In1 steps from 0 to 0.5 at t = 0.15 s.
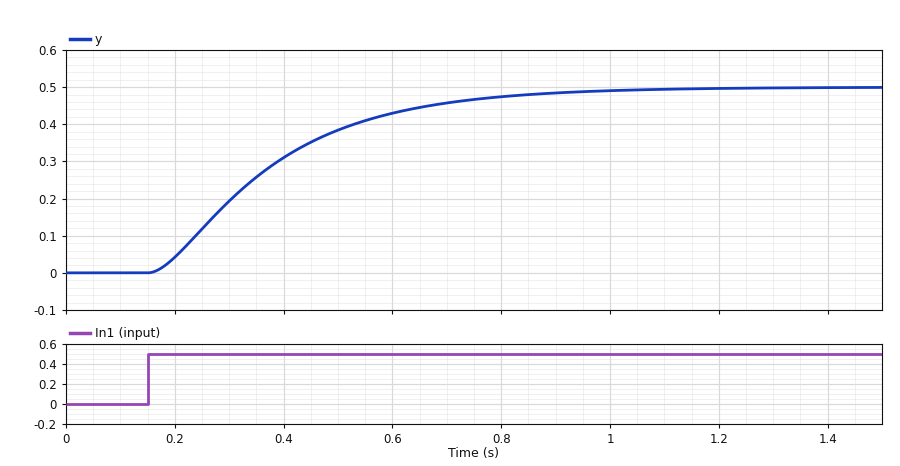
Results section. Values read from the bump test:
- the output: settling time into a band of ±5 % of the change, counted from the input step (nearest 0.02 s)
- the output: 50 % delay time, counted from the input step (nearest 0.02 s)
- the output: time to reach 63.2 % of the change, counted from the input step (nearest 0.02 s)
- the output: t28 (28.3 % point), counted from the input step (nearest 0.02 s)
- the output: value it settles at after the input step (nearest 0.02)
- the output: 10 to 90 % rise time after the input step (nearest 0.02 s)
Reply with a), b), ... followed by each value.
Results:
a) 0.66 s
b) 0.20 s
c) 0.26 s
d) 0.12 s
e) 0.50
f) 0.46 s
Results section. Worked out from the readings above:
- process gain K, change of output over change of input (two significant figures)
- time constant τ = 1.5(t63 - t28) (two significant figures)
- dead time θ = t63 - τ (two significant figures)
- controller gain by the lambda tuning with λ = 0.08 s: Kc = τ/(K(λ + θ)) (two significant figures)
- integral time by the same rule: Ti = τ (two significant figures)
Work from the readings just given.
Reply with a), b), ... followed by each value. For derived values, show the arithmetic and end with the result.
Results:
a) (0.5 - 0) / 0.5 = 1.0
b) 1.5 × (0.26 - 0.12) = 0.21 s
c) 0.26 - 0.21 = 0.050 s
d) 0.21 / (1 × (0.08 + 0.05)) = 1.6
e) 0.21 s
